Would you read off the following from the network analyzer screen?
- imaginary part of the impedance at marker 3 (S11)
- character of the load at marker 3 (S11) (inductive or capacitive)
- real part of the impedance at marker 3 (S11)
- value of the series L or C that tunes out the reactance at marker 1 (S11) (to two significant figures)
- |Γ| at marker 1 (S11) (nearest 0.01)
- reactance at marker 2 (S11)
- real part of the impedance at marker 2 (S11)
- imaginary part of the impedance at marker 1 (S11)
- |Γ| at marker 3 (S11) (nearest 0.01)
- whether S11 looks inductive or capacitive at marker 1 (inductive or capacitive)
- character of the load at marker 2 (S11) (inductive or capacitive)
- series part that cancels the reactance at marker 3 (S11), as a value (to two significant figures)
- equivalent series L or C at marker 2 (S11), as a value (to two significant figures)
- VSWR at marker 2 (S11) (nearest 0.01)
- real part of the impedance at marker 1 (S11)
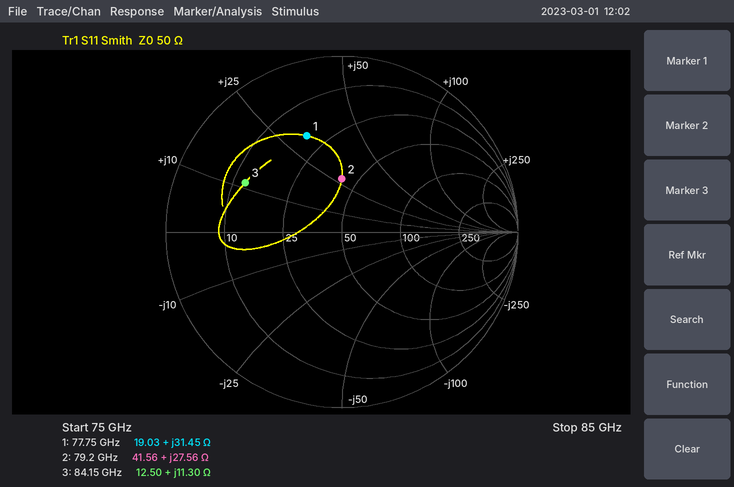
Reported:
+11.30 Ω
inductive
12.50 Ω
65 fF
0.58
+27.56 Ω
41.56 Ω
+31.45 Ω
0.62
inductive
inductive
170 fF
55 pH
1.86
19.03 Ω
